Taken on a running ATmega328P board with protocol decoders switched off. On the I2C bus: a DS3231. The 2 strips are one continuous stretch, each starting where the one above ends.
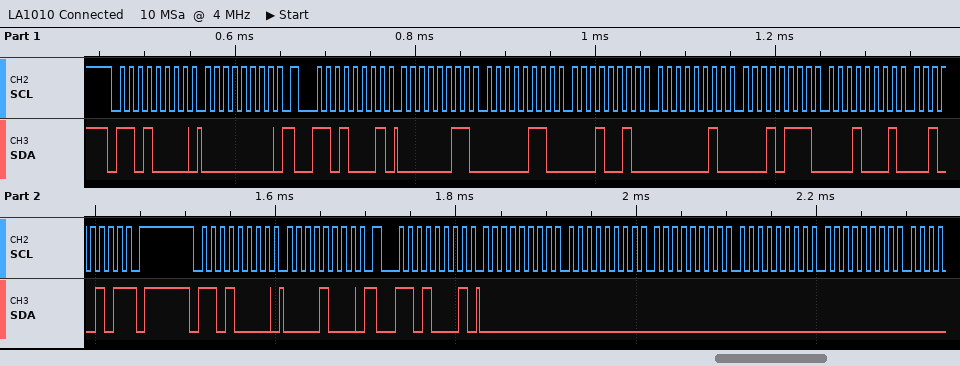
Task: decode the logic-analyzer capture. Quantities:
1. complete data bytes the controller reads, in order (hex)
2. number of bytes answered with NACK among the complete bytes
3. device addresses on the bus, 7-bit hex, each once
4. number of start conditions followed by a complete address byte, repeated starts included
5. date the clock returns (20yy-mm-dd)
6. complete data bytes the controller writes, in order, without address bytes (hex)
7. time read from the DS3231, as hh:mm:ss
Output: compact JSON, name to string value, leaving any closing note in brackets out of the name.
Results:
{"complete data bytes the controller reads, in order": "03 06 12 02 17 11 25 00 00 00 00 00", "number of bytes answered with NACK among the complete bytes": "1", "device addresses on the bus, 7-bit hex, each once": "0x68", "number of start conditions followed by a complete address byte, repeated starts included": "4", "date the clock returns": "2025-11-17", "complete data bytes the controller writes, in order, without address bytes": "00 08", "time read from the DS3231, as hh:mm:ss": "12:06:03"}
